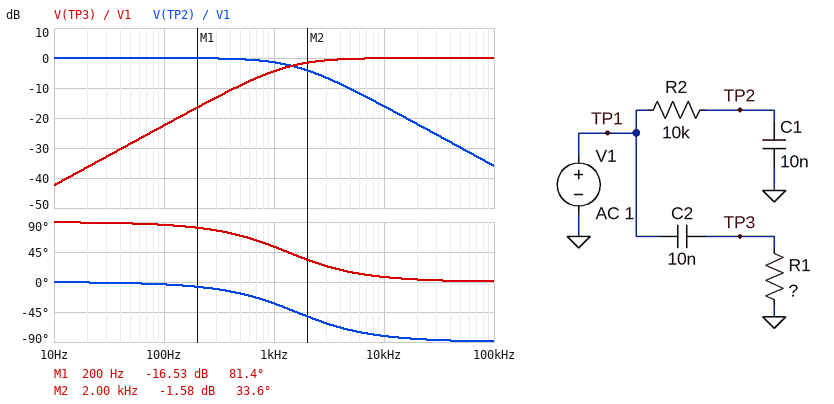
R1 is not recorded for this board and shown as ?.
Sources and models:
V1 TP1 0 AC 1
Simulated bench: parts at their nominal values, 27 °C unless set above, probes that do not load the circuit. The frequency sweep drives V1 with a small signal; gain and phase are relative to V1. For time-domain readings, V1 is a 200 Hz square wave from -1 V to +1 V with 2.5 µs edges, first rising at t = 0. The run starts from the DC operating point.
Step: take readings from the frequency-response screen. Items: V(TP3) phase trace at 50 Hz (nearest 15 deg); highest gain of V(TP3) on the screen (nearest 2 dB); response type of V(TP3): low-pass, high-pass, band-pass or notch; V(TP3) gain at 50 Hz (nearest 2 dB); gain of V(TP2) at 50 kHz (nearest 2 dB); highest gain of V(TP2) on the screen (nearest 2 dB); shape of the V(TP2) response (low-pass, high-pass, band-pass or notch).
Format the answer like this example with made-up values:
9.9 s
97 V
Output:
90 deg
0 dB
high-pass
-28 dB
-30 dB
0 dB
low-pass
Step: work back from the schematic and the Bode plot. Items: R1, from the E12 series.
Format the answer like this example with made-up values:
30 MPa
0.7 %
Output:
12 kΩ
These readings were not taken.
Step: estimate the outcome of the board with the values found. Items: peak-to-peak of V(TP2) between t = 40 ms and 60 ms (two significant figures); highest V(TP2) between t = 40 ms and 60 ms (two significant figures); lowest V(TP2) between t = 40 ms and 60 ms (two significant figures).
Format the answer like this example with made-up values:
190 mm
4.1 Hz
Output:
2.0 V
1.0 V
-1.0 V
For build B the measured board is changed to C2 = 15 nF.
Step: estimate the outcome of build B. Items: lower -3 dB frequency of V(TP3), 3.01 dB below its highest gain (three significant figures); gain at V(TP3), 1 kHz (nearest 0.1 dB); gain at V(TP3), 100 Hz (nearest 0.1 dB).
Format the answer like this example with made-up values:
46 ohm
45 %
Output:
884 Hz
-2.5 dB
-19.0 dB
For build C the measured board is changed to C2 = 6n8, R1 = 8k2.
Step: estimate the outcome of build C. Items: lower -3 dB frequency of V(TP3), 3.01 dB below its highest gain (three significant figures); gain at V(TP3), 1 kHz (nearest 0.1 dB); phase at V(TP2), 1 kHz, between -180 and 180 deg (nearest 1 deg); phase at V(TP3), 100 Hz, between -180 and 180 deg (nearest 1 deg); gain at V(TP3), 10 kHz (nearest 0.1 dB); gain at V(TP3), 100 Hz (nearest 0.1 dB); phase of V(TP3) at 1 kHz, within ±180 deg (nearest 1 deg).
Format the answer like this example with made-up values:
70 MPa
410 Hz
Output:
2.85 kHz
-9.6 dB
-32 deg
88 deg
-0.3 dB
-29.1 dB
71 deg
